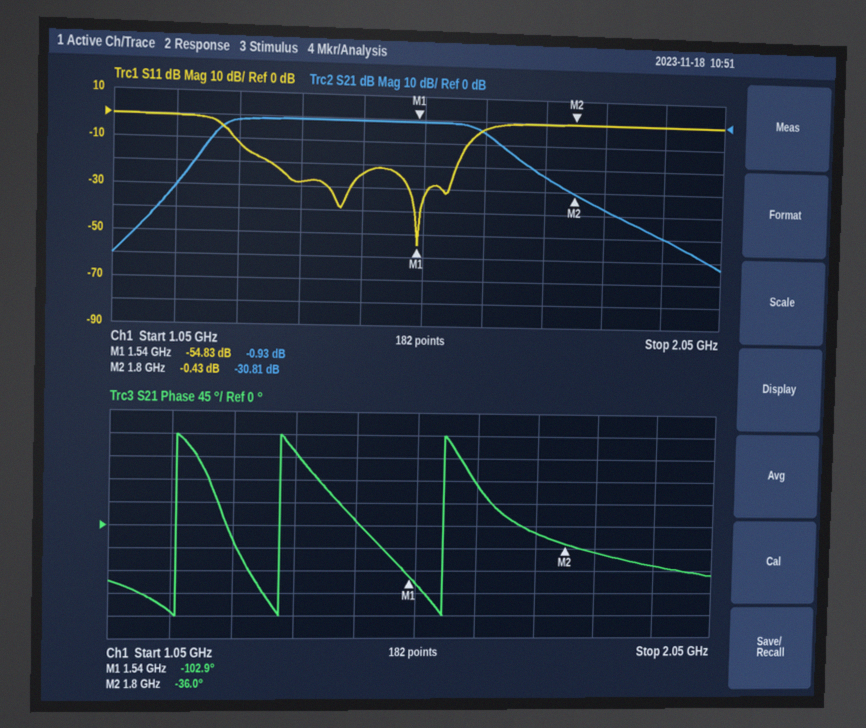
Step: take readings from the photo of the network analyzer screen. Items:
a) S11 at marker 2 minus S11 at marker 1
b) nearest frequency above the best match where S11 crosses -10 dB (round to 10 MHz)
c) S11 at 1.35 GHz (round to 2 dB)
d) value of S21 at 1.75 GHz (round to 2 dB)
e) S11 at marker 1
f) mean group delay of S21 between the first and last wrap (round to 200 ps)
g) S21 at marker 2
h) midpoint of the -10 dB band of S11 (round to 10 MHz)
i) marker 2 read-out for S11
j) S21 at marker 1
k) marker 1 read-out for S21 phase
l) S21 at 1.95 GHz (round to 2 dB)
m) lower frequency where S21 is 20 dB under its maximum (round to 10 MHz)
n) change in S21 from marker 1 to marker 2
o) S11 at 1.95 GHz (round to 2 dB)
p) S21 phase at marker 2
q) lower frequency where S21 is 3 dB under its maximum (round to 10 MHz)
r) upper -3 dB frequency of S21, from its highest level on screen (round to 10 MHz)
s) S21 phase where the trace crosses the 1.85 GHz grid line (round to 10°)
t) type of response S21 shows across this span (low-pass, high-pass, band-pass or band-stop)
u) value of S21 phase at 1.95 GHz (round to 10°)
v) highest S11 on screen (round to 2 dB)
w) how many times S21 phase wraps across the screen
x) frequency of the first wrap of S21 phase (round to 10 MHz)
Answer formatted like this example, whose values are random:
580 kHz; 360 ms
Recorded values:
54.40 dB; 1.62 GHz; -28 dB; -24 dB; -54.83 dB; 4.6 ns; -30.81 dB; 1.43 GHz; -0.43 dB; -0.93 dB; -102.9°; -50 dB; 1.18 GHz; -29.88 dB; 0 dB; -36.0°; 1.23 GHz; 1.64 GHz; -50°; band-pass; -80°; 0 dB; 3; 1.16 GHz
